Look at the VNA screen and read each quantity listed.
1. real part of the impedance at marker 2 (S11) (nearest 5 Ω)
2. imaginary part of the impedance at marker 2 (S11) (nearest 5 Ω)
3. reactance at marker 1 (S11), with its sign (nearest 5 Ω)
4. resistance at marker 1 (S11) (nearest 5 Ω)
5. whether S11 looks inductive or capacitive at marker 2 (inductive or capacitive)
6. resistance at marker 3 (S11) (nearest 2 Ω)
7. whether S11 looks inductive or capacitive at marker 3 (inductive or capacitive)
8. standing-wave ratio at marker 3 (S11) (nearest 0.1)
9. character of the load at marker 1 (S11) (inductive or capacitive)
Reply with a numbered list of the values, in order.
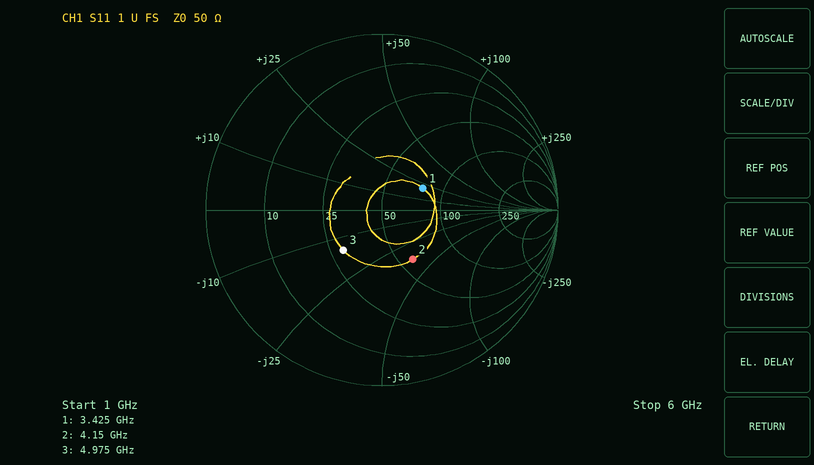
1. 60 Ω
2. -35 Ω
3. +20 Ω
4. 75 Ω
5. capacitive
6. 30 Ω
7. capacitive
8. 1.9
9. inductive
